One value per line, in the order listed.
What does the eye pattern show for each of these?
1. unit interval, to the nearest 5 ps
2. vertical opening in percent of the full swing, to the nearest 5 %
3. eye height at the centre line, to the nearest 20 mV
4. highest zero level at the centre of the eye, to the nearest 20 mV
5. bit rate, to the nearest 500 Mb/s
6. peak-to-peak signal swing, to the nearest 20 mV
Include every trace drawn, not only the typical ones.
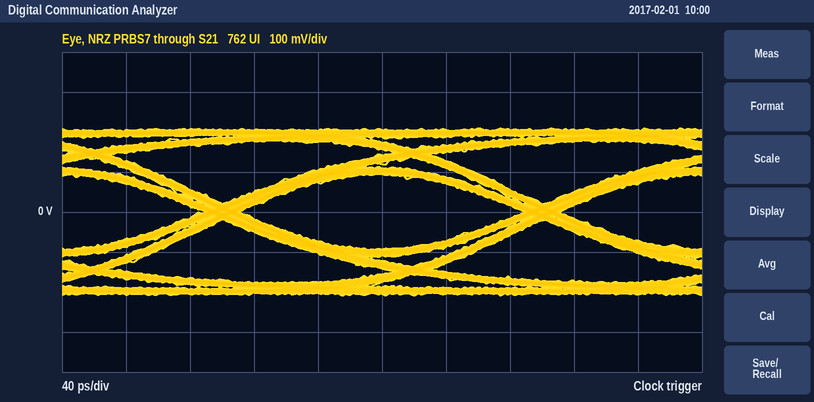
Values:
200 ps
45 %
180 mV
-100 mV
5.0 Gb/s
420 mV
